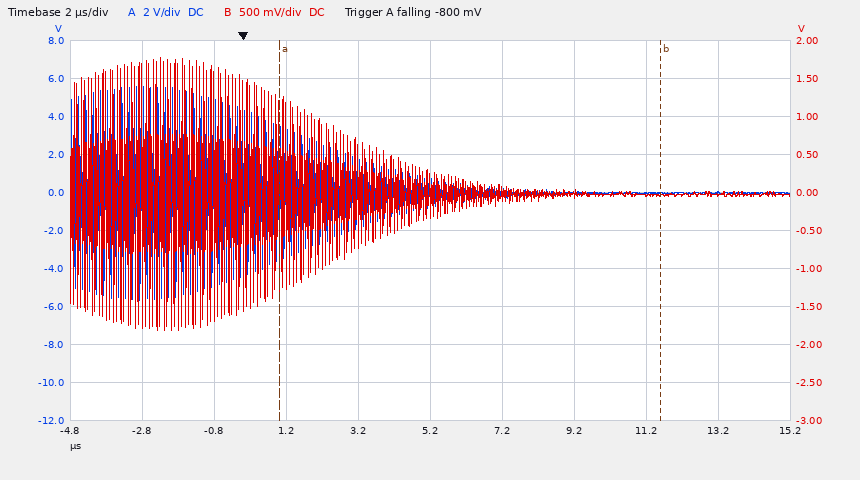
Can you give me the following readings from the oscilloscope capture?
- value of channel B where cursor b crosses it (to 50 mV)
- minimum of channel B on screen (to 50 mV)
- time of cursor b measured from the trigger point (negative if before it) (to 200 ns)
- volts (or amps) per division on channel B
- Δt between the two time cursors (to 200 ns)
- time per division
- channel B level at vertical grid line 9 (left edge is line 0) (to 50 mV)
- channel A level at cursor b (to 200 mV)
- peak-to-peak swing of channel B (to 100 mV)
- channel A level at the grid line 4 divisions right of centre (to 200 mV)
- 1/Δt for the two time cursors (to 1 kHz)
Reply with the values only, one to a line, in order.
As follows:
-50 mV
-1.80 V
+11.6 µs
500 mV
10.6 µs
2 µs
-50 mV
0.0 V
3.60 V
0.0 V
94 kHz
